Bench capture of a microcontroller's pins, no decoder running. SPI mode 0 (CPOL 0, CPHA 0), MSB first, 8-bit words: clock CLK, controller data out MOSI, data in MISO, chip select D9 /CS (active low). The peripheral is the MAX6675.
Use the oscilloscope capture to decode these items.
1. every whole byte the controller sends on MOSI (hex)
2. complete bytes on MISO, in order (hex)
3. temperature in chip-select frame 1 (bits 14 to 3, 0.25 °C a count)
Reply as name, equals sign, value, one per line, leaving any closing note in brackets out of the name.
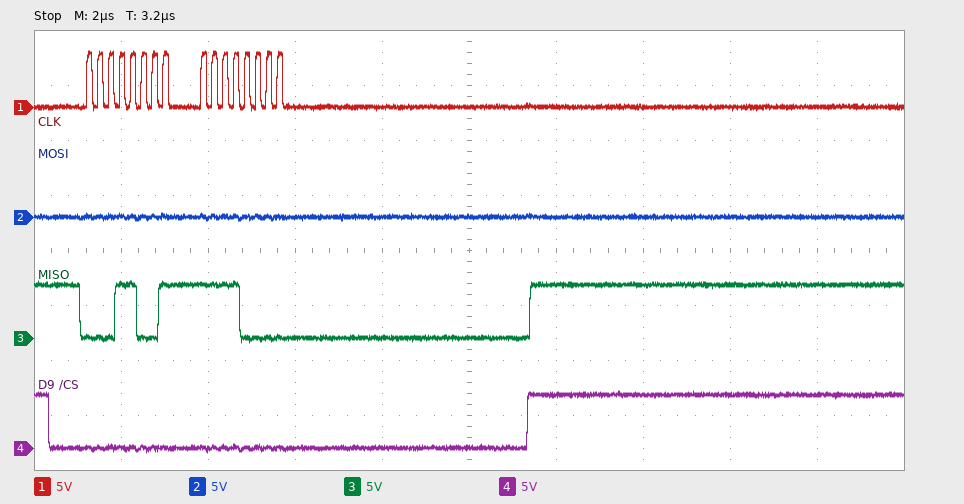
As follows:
every whole byte the controller sends on MOSI = 00 00
complete bytes on MISO, in order = 19 F0
temperature in chip-select frame 1 = 207.50 °C
